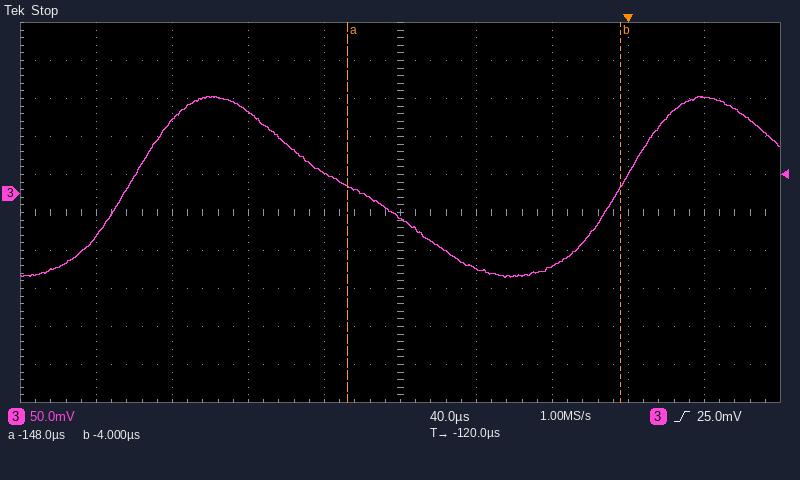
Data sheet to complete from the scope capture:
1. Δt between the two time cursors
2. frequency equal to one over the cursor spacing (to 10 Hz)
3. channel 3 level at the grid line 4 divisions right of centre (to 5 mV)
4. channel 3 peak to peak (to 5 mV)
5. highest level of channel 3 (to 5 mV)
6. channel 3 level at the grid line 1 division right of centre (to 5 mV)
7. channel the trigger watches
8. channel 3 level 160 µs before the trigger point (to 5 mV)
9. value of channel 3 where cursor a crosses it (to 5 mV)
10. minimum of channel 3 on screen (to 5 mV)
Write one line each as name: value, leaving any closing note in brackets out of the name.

Δt between the two time cursors: 144 µs
frequency equal to one over the cursor spacing: 6.94 kHz
channel 3 level at the grid line 4 divisions right of centre: 125 mV
channel 3 peak to peak: 240 mV
highest level of channel 3: 130 mV
channel 3 level at the grid line 1 division right of centre: -100 mV
channel the trigger watches: channel 3
channel 3 level 160 µs before the trigger point: 25 mV
value of channel 3 where cursor a crosses it: 10 mV
minimum of channel 3 on screen: -110 mV
